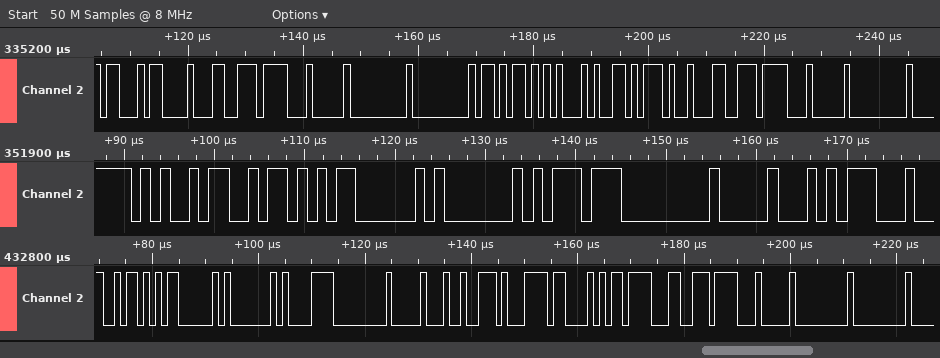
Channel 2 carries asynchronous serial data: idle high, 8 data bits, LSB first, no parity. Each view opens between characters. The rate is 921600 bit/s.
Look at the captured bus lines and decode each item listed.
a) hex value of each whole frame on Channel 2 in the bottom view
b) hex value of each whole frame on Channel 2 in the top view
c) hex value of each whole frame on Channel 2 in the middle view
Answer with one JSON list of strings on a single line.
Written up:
["5A, 03, 01, E1, 00, 10, 72, BC, A8, 8F, EE, 04, 00, 00", "A3, 88, EE, 04, 00, 00, 6B, 45, D6, 89, EE, 04, 00", "A5, 5A, 03, 01, DD, 00, 10, 1D"]
